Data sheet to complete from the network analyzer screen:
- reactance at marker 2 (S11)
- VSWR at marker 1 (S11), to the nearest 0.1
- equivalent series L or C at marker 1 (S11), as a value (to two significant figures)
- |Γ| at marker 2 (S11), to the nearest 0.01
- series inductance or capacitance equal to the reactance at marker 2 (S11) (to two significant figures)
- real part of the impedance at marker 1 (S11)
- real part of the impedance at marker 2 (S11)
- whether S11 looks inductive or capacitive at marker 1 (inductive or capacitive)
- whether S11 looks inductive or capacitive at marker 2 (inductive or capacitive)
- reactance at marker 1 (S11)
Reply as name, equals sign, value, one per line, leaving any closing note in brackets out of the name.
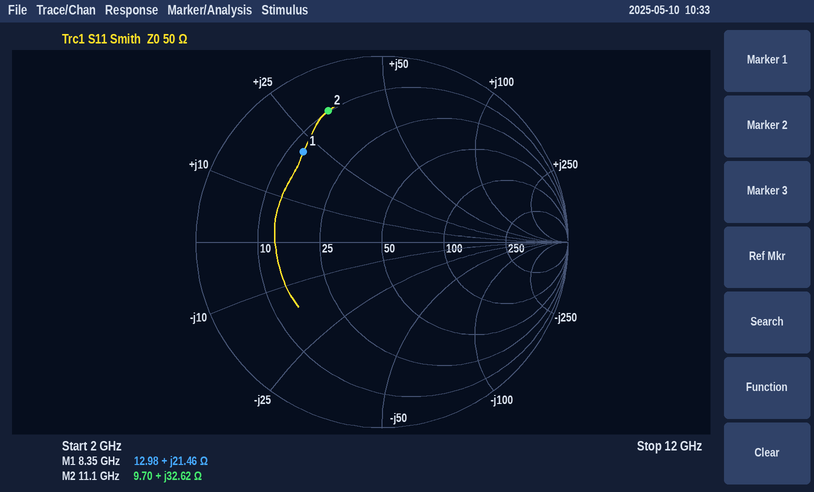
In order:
reactance at marker 2 = +32.62 Ω
VSWR at marker 1 (S11), to the nearest 0.1 = 4.6
equivalent series L or C at marker 1 (S11), as a value = 410 pH
|Γ| at marker 2 (S11), to the nearest 0.01 = 0.76
series inductance or capacitance equal to the reactance at marker 2 (S11) = 470 pH
real part of the impedance at marker 1 = 12.98 Ω
real part of the impedance at marker 2 = 9.70 Ω
whether S11 looks inductive or capacitive at marker 1 = inductive
whether S11 looks inductive or capacitive at marker 2 = inductive
reactance at marker 1 = +21.46 Ω
